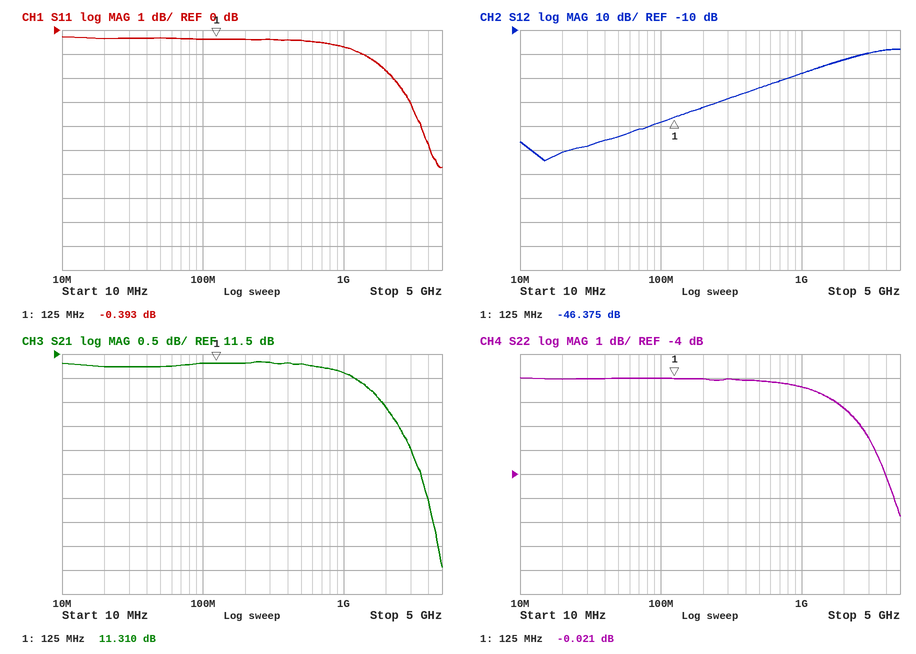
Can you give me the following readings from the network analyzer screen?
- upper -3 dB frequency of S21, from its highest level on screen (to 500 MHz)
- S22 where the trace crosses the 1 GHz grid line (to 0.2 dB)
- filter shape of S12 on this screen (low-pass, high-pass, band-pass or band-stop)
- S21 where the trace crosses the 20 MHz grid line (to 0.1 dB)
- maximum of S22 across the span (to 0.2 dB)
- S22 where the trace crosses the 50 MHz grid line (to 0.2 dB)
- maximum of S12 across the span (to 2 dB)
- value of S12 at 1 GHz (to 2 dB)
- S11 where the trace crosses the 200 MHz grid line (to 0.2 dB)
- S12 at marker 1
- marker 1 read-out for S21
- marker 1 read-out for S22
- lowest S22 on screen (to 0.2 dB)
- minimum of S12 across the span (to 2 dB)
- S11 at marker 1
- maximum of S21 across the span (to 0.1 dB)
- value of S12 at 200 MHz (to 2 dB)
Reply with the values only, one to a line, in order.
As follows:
4.0 GHz
-0.4 dB
high-pass
11.2 dB
0.0 dB
0.0 dB
-18 dB
-28 dB
-0.4 dB
-46.375 dB
11.310 dB
-0.021 dB
-5.8 dB
-64 dB
-0.393 dB
11.3 dB
-42 dB
